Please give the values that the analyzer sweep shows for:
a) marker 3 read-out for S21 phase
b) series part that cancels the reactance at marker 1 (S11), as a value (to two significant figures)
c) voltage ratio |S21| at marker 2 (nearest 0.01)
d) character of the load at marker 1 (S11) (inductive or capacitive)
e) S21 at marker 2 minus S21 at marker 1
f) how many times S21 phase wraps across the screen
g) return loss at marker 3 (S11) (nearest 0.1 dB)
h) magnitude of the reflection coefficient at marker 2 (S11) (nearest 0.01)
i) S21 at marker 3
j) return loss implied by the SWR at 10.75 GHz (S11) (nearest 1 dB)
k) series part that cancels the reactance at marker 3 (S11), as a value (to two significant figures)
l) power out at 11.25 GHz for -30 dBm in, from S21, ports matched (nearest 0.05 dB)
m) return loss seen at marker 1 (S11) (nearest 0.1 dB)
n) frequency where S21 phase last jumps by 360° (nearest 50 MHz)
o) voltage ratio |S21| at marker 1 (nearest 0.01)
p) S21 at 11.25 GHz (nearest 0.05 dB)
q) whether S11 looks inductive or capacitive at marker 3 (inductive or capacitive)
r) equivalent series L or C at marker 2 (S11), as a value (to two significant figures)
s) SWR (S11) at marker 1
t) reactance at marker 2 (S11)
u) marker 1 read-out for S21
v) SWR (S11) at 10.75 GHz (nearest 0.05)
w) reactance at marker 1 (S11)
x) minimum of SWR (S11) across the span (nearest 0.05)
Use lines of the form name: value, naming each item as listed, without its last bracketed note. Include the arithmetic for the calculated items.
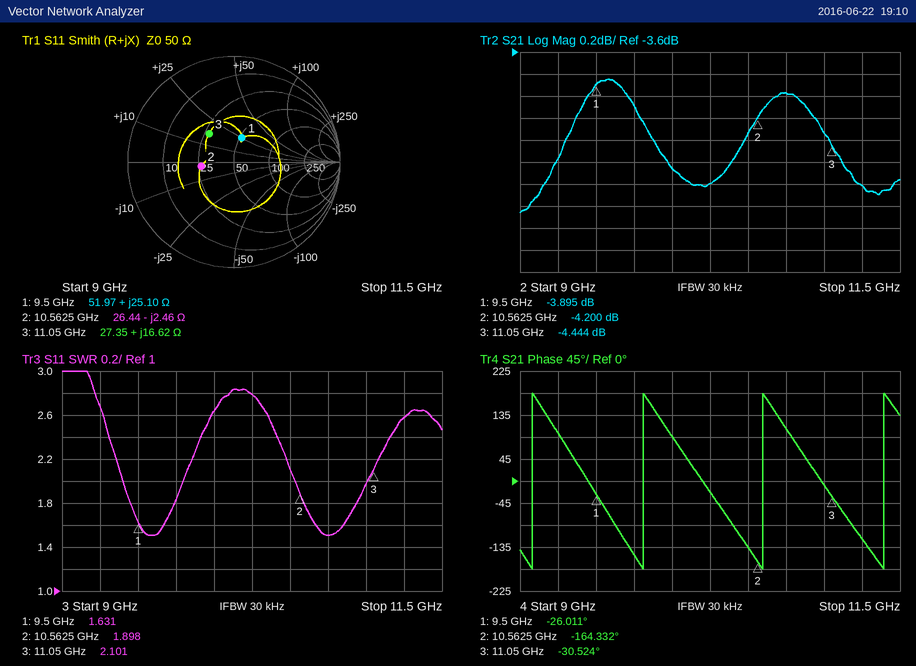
marker 3 read-out for S21 phase: -30.524°
series part that cancels the reactance at marker 1 (S11), as a value: C = 1/(2π × 9.5 GHz × 25.1 Ω) ≈ 667 fF, so 670 fF to two significant figures
voltage ratio |S21| at marker 2: 10^(-4.2/20) ≈ 0.62
character of the load at marker 1 (S11): inductive
S21 at marker 2 minus S21 at marker 1: -4.2 − (-3.895) = -0.305 dB
how many times S21 phase wraps across the screen: 4
return loss at marker 3 (S11): 9.0 dB
magnitude of the reflection coefficient at marker 2 (S11): 0.31
S21 at marker 3: -4.444 dB
return loss implied by the SWR at 10.75 GHz (S11): −20 log10((1.5 − 1)/(1.5 + 1)) ≈ 14 dB
series part that cancels the reactance at marker 3 (S11), as a value: C = 1/(2π × 11.05 GHz × 16.62 Ω) ≈ 867 fF, so 870 fF to two significant figures
power out at 11.25 GHz for -30 dBm in, from S21, ports matched: -30 dBm + (-4.80 dB) = -34.80 dBm
return loss seen at marker 1 (S11): 12.4 dB
frequency where S21 phase last jumps by 360°: 11.40 GHz
voltage ratio |S21| at marker 1: 10^(-3.895/20) ≈ 0.64
S21 at 11.25 GHz: -4.80 dB
whether S11 looks inductive or capacitive at marker 3: inductive
equivalent series L or C at marker 2 (S11), as a value: C = 1/(2π × 10.5625 GHz × 2.46 Ω) ≈ 6.1 pF
SWR (S11) at marker 1: 1.631
reactance at marker 2: -2.46 Ω
marker 1 read-out for S21: -3.895 dB
SWR (S11) at 10.75 GHz: 1.50
reactance at marker 1: +25.10 Ω
minimum of SWR (S11) across the span: 1.50
